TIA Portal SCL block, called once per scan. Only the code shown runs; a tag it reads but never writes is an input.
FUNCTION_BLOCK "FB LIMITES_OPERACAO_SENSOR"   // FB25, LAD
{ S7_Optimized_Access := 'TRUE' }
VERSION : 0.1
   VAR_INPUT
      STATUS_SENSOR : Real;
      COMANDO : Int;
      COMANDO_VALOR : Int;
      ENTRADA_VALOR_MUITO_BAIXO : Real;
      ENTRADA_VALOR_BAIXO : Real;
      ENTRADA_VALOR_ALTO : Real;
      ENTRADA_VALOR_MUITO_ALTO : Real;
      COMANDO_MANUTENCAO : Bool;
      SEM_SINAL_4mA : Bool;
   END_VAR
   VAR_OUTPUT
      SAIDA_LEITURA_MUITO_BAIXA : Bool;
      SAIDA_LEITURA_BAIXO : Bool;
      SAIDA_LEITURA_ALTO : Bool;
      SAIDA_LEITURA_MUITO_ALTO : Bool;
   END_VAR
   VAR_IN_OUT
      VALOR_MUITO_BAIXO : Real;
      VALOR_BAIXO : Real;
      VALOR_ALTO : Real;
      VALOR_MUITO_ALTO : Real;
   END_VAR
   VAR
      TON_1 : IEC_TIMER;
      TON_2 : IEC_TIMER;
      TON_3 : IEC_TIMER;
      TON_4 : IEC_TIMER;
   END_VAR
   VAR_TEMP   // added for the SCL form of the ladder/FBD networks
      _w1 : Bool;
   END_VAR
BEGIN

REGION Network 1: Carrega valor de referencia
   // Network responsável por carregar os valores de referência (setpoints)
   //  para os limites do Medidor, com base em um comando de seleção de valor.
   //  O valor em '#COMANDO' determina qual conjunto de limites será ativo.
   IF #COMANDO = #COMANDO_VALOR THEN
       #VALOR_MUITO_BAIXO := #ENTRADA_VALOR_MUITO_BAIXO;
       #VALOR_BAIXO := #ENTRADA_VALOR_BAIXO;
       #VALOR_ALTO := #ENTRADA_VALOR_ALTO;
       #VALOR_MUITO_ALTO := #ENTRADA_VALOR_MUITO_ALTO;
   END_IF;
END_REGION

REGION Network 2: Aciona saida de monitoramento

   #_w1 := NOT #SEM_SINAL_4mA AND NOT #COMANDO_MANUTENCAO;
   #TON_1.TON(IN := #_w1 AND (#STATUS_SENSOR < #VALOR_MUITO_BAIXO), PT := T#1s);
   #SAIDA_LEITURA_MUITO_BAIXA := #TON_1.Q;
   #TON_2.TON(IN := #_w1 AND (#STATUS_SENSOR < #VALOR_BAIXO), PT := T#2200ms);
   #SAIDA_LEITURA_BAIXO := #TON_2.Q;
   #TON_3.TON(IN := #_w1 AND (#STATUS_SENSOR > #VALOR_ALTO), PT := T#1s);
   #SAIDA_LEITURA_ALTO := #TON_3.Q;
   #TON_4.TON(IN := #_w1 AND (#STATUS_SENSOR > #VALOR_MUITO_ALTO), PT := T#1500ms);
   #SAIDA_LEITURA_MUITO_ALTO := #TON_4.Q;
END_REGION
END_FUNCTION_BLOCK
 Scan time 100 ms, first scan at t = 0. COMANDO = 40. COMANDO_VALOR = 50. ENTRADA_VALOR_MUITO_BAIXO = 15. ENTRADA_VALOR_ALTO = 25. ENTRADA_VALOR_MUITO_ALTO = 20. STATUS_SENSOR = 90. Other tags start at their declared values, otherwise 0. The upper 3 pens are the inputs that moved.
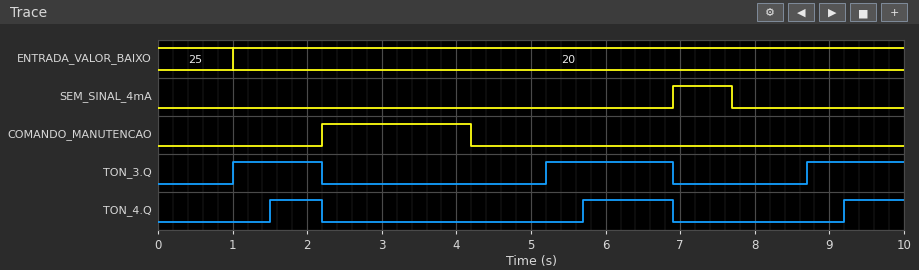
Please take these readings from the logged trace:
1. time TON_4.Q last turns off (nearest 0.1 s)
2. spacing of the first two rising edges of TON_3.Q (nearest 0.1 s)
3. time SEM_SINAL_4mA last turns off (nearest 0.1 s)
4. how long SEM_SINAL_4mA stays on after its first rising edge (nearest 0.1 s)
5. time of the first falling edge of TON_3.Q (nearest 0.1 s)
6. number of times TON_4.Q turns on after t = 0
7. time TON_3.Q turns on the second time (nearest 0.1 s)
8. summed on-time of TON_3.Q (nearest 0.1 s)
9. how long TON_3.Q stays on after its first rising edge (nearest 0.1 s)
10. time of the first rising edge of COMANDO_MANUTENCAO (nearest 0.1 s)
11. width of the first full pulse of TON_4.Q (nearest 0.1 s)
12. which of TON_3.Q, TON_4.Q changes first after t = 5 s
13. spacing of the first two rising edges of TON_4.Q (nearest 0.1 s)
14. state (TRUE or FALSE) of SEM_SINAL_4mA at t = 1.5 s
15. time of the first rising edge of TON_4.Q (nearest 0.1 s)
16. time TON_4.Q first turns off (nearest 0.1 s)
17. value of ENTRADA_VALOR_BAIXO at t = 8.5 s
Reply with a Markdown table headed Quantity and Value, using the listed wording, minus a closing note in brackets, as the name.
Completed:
| Quantity | Value |
|---|---|
| time TON_4.Q last turns off | 6.9 s |
| spacing of the first two rising edges of TON_3.Q | 4.2 s |
| time SEM_SINAL_4mA last turns off | 7.7 s |
| how long SEM_SINAL_4mA stays on after its first rising edge | 0.8 s |
| time of the first falling edge of TON_3.Q | 2.2 s |
| number of times TON_4.Q turns on after t = 0 | 3 |
| time TON_3.Q turns on the second time | 5.2 s |
| summed on-time of TON_3.Q | 4.2 s |
| how long TON_3.Q stays on after its first rising edge | 1.2 s |
| time of the first rising edge of COMANDO_MANUTENCAO | 2.2 s |
| width of the first full pulse of TON_4.Q | 0.7 s |
| which of TON_3.Q, TON_4.Q changes first after t = 5 s | TON_3.Q |
| spacing of the first two rising edges of TON_4.Q | 4.2 s |
| state (TRUE or FALSE) of SEM_SINAL_4mA at t = 1.5 s | FALSE |
| time of the first rising edge of TON_4.Q | 1.5 s |
| time TON_4.Q first turns off | 2.2 s |
| value of ENTRADA_VALOR_BAIXO at t = 8.5 s | 20 |
